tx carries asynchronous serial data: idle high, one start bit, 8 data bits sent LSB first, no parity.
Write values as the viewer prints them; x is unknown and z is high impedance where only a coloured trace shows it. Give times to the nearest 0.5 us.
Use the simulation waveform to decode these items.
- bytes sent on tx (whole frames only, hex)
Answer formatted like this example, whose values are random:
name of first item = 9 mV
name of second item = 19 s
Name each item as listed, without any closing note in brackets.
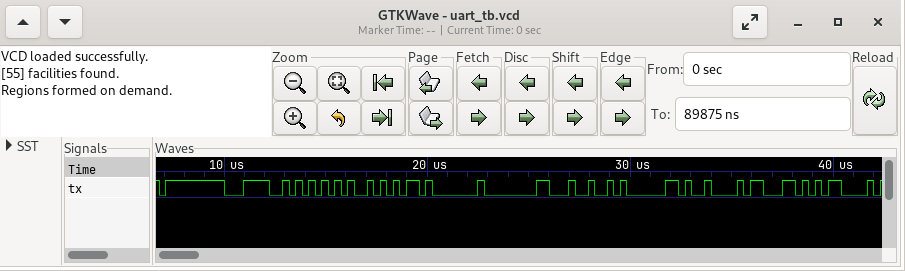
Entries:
bytes sent on tx = FF, 3C, 55, AA, 01, 80, 24, 81, 09, 63, 0D
